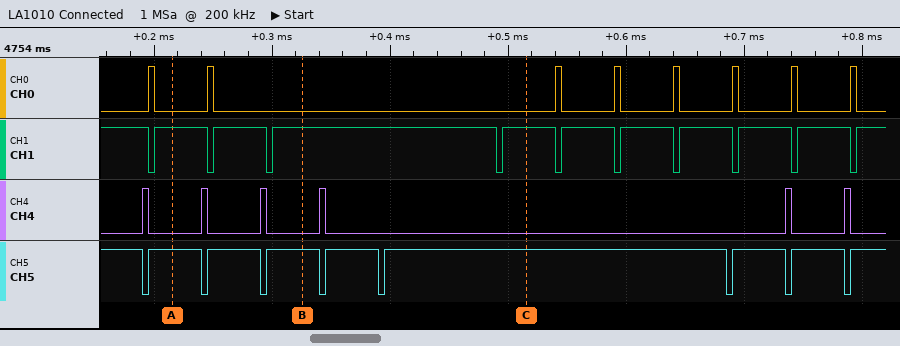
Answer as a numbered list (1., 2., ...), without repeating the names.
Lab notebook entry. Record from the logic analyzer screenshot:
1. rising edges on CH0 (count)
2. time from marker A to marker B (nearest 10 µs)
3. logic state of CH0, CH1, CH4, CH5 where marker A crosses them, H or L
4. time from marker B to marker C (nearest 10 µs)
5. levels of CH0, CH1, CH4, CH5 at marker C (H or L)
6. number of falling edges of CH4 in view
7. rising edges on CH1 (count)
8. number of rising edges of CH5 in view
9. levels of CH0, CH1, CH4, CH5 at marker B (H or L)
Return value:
1. 8
2. 110 µs
3. CH0=L, CH1=H, CH4=L, CH5=H
4. 190 µs
5. CH0=L, CH1=H, CH4=L, CH5=H
6. 6
7. 10
8. 8
9. CH0=L, CH1=H, CH4=L, CH5=H
